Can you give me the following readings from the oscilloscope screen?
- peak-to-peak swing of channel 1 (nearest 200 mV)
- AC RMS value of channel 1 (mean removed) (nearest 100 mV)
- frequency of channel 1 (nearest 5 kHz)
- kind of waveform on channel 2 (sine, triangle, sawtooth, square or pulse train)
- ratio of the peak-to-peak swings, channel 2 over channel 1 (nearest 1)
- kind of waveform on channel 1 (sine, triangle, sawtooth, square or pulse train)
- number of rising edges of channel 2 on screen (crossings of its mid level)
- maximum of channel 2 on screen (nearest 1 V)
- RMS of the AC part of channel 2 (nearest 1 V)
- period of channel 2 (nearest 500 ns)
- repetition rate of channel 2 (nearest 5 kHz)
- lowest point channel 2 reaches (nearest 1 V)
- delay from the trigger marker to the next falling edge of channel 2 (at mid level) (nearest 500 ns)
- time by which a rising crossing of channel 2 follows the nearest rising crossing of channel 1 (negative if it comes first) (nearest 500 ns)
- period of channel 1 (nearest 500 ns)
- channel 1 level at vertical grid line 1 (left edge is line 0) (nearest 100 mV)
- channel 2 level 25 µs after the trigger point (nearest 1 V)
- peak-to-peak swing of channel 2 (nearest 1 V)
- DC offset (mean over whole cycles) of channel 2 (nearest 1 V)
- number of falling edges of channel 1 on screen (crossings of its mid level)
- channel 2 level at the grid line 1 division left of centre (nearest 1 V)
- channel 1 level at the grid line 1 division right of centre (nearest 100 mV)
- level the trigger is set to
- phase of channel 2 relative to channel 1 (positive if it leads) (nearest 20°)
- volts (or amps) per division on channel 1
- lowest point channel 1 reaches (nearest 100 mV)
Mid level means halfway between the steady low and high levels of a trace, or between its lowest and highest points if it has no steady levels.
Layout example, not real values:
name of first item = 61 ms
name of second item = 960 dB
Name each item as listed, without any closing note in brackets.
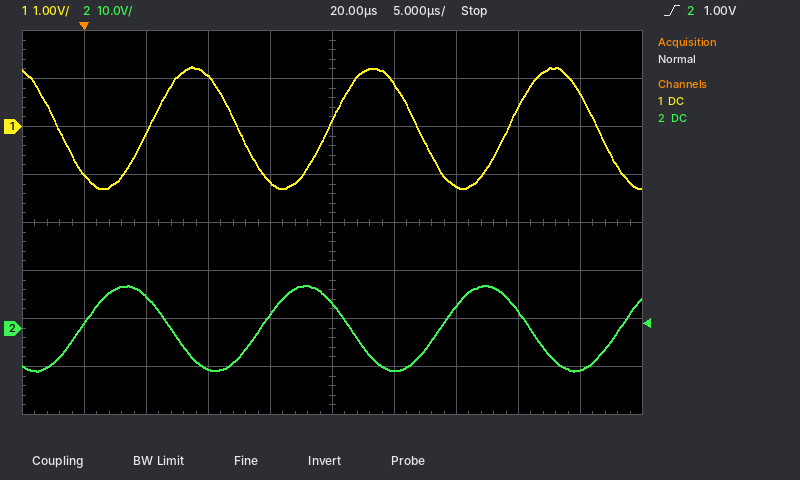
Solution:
peak-to-peak swing of channel 1 = 2.6 V
AC RMS value of channel 1 (mean removed) = 900 mV
frequency of channel 1 = 70 kHz
kind of waveform on channel 2 = sine
ratio of the peak-to-peak swings, channel 2 over channel 1 = 7
kind of waveform on channel 1 = sine
number of rising edges of channel 2 on screen = 4
maximum of channel 2 on screen = 9 V
RMS of the AC part of channel 2 = 6 V
period of channel 2 = 14.5 µs
repetition rate of channel 2 = 70 kHz
lowest point channel 2 reaches = -9 V
delay from the trigger marker to the next falling edge of channel 2 (at mid level) = 7.0 µs
time by which a rising crossing of channel 2 follows the nearest rising crossing of channel 1 (negative if it comes first) = -5.5 µs
period of channel 1 = 14.5 µs
channel 1 level at vertical grid line 1 (left edge is line 0) = -1.0 V
channel 2 level 25 µs after the trigger point = -9 V
peak-to-peak swing of channel 2 = 18 V
DC offset (mean over whole cycles) of channel 2 = 0 V
number of falling edges of channel 1 on screen = 4
channel 2 level at the grid line 1 division left of centre = 3 V
channel 1 level at the grid line 1 division right of centre = 900 mV
level the trigger is set to = 1.00 V
phase of channel 2 relative to channel 1 (positive if it leads) = +140°
volts (or amps) per division on channel 1 = 1 V
lowest point channel 1 reaches = -1.3 V
